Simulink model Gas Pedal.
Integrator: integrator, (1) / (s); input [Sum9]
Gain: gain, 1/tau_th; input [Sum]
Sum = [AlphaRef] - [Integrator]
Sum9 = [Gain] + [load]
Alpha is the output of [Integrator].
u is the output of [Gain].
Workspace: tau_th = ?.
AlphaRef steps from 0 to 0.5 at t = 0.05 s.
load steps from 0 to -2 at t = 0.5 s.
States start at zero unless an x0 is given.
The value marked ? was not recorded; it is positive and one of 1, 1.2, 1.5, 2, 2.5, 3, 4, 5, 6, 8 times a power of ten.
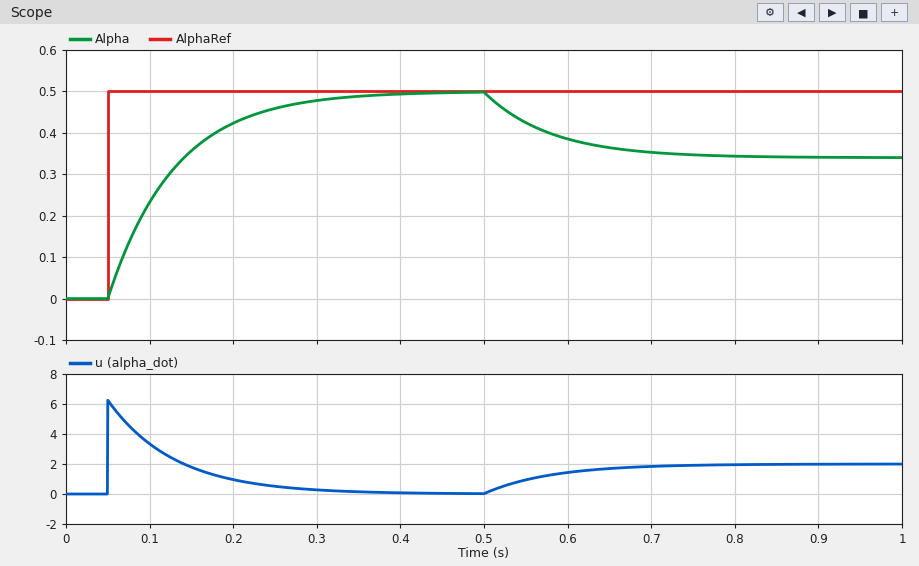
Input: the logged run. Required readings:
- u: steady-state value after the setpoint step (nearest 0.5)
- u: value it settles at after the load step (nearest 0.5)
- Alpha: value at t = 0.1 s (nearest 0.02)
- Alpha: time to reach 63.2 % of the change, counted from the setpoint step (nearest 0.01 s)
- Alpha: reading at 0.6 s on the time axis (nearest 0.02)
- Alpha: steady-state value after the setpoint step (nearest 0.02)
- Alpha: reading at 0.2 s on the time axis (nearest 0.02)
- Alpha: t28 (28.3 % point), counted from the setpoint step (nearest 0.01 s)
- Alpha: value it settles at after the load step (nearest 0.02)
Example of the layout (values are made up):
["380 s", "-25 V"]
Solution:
["0.0", "2.0", "0.24", "0.08 s", "0.38", "0.50", "0.42", "0.03 s", "0.34"]
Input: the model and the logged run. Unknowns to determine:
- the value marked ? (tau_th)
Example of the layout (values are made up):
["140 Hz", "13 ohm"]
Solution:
["0.08"]
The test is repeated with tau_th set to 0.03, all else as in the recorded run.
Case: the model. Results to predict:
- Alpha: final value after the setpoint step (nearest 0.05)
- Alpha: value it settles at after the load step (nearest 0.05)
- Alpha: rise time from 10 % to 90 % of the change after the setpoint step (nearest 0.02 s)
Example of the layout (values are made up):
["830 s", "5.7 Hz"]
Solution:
["0.50", "0.45", "0.06 s"]
